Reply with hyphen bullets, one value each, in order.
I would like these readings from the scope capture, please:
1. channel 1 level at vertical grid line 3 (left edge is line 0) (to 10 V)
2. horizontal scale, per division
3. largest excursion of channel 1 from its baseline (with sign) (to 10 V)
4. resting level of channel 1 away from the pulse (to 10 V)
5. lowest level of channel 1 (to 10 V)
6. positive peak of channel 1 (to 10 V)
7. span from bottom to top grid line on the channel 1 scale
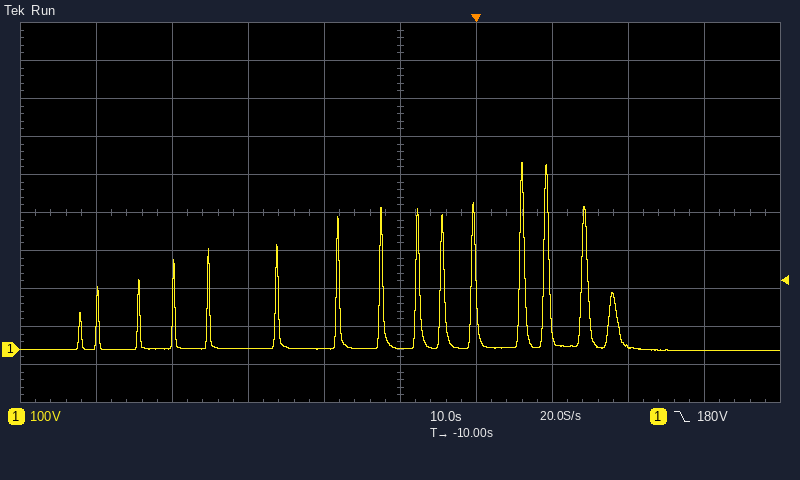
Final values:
- 0 V
- 10 s
- +490 V
- 0 V
- 0 V
- 490 V
- 1 kV
